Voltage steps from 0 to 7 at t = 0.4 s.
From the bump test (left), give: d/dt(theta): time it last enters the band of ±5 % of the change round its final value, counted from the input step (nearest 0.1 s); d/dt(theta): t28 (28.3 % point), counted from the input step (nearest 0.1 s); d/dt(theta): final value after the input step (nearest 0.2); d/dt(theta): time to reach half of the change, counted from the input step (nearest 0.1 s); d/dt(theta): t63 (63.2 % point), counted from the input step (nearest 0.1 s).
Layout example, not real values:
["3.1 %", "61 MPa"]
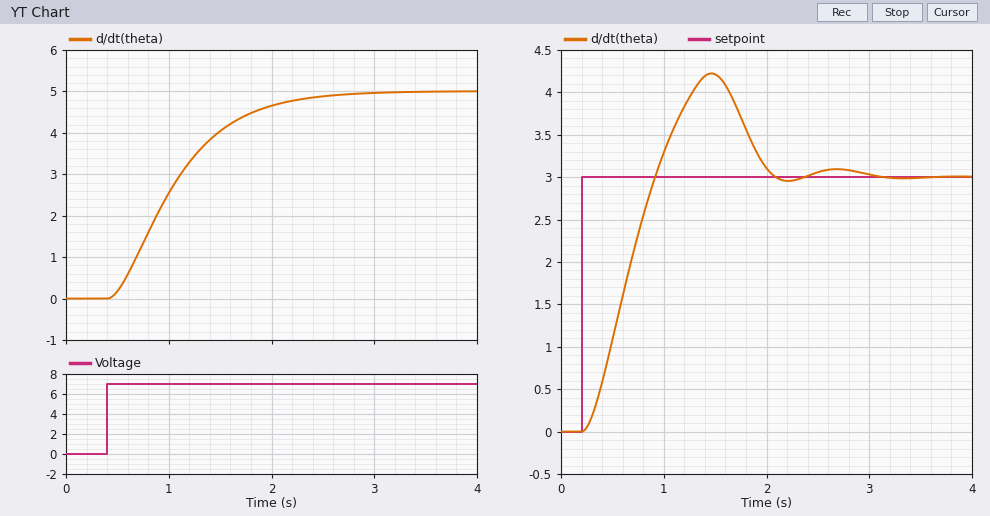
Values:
["1.8 s", "0.4 s", "5.0", "0.6 s", "0.8 s"]
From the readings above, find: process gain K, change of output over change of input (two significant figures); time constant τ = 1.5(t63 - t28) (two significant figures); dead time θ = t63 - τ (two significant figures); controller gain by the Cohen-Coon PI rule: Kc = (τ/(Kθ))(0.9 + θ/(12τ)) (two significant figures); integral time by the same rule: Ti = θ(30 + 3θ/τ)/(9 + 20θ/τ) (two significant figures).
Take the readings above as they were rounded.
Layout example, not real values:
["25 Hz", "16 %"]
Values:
["0.71", "0.60 s", "0.20 s", "3.9", "0.40 s"]
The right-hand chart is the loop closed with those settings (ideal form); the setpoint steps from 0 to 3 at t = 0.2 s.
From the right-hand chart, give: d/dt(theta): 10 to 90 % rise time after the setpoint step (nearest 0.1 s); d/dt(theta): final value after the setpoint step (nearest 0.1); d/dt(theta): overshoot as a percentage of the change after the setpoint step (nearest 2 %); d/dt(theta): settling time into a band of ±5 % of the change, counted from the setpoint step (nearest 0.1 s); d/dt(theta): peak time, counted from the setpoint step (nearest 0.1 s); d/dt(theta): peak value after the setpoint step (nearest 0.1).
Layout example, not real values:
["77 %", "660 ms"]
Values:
["0.5 s", "3.0", "40 %", "1.8 s", "1.3 s", "4.2"]
